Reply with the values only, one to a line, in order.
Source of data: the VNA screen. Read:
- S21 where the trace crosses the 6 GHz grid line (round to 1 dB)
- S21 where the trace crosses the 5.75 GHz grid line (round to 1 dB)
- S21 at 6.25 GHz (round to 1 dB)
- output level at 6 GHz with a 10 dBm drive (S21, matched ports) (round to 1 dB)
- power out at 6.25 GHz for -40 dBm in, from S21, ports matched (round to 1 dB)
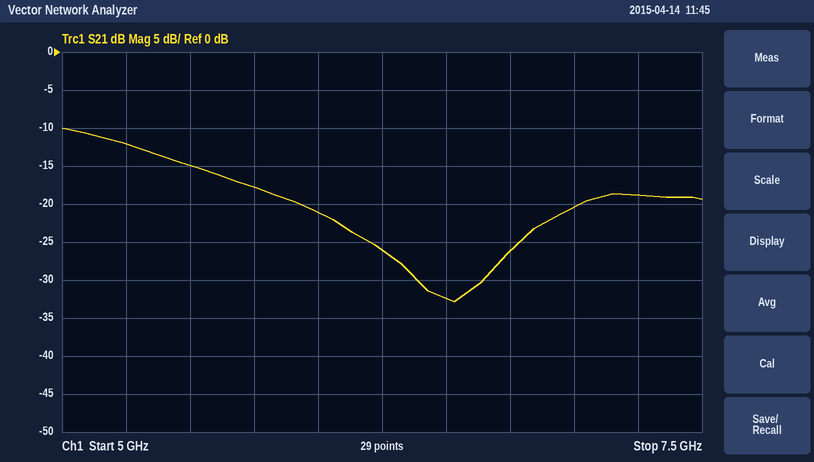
-21 dB
-18 dB
-26 dB
-11 dBm
-66 dBm
